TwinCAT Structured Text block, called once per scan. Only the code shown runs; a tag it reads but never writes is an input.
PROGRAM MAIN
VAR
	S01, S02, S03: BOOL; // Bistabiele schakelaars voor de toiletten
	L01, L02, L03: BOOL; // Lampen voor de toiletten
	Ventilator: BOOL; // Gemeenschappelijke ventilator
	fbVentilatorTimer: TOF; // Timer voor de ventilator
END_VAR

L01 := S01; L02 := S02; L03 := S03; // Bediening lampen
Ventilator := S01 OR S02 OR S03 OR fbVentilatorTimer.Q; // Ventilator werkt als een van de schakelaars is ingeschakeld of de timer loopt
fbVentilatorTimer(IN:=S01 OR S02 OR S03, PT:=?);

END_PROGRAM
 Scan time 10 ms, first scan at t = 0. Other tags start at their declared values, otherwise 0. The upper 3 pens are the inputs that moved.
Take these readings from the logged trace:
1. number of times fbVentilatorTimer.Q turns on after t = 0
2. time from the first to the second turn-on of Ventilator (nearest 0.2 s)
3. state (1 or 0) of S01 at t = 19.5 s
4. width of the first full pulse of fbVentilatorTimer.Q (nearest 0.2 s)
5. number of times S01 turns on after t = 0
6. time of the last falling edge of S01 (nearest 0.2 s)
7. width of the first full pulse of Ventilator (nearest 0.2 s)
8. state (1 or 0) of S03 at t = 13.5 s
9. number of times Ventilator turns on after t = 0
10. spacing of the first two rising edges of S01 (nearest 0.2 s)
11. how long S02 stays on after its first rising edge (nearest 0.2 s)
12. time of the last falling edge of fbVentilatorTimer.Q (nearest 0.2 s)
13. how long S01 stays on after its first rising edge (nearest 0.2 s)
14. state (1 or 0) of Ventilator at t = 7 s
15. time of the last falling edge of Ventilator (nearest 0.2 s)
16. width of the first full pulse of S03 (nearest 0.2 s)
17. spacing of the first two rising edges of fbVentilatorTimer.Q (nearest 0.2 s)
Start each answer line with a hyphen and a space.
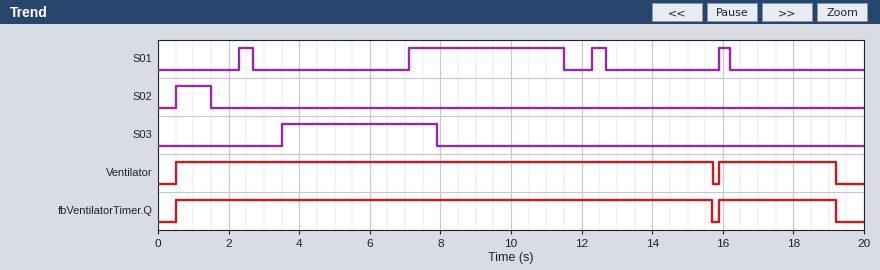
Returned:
- 2
- 15.4 s
- 0
- 15.2 s
- 4
- 16.2 s
- 15.2 s
- 0
- 2
- 4.8 s
- 1.0 s
- 19.2 s
- 0.4 s
- 1
- 19.2 s
- 4.4 s
- 15.4 s
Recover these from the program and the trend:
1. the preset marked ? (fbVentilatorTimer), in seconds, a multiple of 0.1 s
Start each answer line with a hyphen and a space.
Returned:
- 3.0 s
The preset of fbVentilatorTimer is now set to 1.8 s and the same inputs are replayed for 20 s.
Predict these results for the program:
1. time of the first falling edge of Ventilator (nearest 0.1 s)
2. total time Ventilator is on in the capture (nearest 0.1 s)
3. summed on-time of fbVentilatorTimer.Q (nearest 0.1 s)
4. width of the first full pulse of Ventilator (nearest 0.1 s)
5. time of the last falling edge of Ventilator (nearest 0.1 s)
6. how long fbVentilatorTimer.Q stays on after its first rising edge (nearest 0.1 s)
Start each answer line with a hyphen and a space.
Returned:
- 14.5 s
- 16.1 s
- 16.1 s
- 14.0 s
- 18.0 s
- 14.0 s
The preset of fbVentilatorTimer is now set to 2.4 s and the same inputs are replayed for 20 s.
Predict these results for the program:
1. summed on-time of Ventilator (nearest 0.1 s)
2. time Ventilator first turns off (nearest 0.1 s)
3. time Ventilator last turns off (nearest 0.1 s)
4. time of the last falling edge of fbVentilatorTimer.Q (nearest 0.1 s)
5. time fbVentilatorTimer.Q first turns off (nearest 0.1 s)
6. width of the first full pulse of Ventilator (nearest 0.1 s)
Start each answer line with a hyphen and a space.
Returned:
- 17.3 s
- 15.1 s
- 18.6 s
- 18.6 s
- 15.1 s
- 14.6 s
